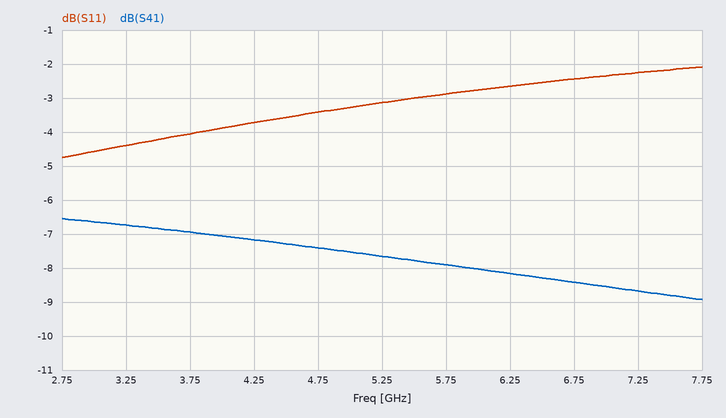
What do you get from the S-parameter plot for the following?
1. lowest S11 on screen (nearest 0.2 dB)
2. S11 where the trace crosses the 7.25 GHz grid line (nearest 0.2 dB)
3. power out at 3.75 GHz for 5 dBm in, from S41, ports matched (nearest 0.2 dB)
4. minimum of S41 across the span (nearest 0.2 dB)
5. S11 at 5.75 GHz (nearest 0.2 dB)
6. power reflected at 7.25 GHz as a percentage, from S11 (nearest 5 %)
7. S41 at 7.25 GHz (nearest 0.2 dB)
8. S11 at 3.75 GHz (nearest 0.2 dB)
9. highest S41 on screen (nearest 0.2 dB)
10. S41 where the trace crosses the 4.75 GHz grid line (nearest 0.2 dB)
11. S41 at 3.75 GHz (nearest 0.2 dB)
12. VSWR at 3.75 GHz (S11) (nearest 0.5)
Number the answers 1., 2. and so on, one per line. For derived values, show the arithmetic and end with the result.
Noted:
1. -4.8 dB
2. -2.2 dB
3. 5 dBm + (-7.0 dB) = -2.0 dBm
4. -9.0 dB
5. -2.8 dB
6. 10^(-2.2/10) ≈ 60 %
7. -8.6 dB
8. -4.0 dB
9. -6.6 dB
10. -7.4 dB
11. -7.0 dB
12. |Γ| = 10^(-4/20) = 0.6310; VSWR = (1 + 0.6310)/(1 − 0.6310) ≈ 4.42, so 4.5 to the nearest 0.5
